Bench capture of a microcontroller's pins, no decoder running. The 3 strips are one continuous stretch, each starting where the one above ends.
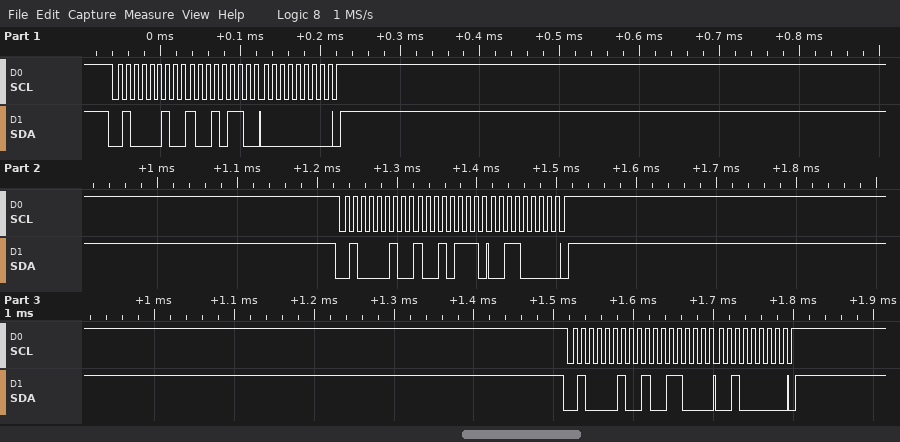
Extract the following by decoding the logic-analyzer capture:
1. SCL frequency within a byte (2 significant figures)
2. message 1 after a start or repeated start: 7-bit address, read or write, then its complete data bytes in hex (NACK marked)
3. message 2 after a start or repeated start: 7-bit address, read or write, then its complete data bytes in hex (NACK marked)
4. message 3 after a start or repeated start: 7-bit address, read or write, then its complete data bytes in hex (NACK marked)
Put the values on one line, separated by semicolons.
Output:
100 kHz; 0x21 write: 96 00; 0x21 write: 97 30; 0x21 write: 98 20
